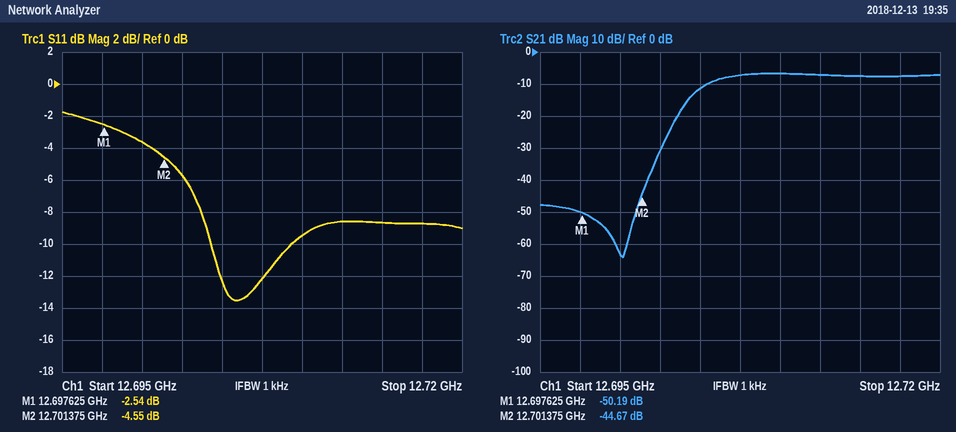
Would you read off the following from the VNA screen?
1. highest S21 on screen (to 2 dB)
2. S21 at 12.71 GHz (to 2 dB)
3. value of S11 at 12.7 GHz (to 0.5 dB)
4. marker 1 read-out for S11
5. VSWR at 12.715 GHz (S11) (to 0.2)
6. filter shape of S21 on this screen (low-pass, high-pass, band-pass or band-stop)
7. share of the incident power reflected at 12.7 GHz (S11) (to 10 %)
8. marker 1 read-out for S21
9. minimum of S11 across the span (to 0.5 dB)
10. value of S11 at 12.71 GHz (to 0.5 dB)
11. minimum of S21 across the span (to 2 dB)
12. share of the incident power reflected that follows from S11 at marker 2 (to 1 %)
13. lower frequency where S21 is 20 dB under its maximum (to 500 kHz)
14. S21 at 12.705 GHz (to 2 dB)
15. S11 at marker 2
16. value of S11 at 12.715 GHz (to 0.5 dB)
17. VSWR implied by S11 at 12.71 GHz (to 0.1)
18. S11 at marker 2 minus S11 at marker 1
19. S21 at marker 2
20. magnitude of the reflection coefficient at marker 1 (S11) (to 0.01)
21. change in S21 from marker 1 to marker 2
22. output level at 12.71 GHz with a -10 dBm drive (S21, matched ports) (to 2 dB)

-6 dB
-6 dB
-3.5 dB
-2.54 dB
2.2
high-pass
40 %
-50.19 dB
-13.5 dB
-9.5 dB
-64 dB
35 %
12.7030 GHz
-12 dB
-4.55 dB
-8.5 dB
2.0
-2.01 dB
-44.67 dB
0.75
5.52 dB
-16 dBm
